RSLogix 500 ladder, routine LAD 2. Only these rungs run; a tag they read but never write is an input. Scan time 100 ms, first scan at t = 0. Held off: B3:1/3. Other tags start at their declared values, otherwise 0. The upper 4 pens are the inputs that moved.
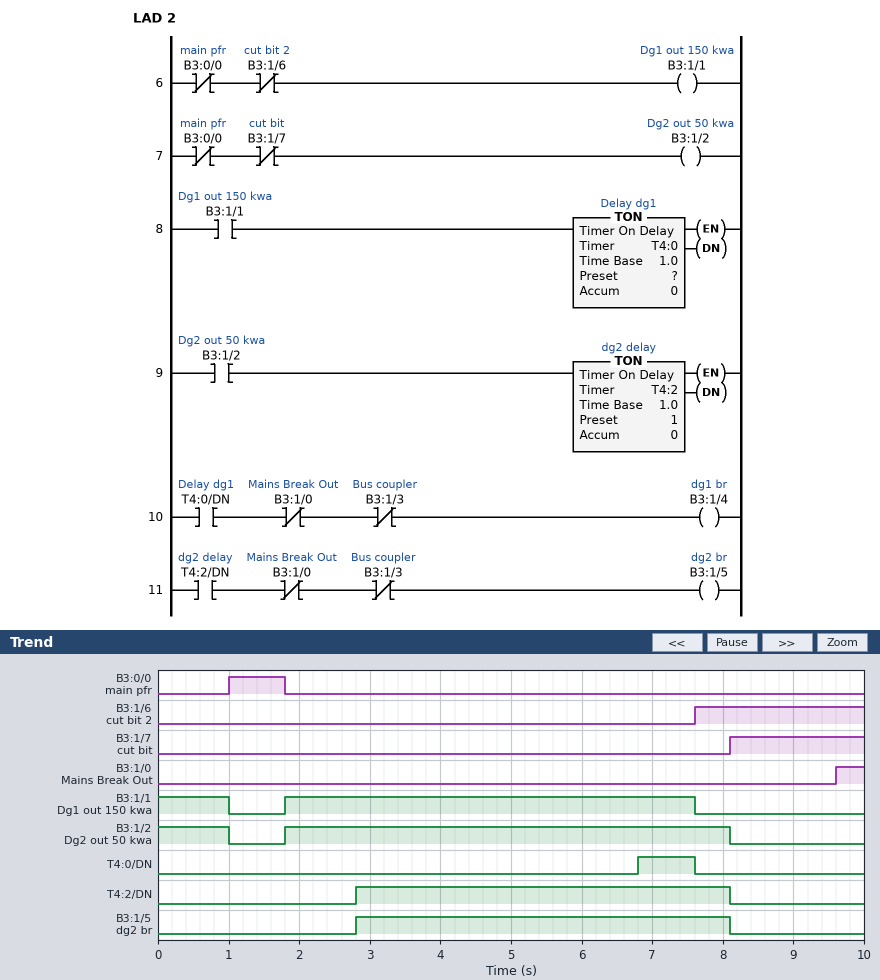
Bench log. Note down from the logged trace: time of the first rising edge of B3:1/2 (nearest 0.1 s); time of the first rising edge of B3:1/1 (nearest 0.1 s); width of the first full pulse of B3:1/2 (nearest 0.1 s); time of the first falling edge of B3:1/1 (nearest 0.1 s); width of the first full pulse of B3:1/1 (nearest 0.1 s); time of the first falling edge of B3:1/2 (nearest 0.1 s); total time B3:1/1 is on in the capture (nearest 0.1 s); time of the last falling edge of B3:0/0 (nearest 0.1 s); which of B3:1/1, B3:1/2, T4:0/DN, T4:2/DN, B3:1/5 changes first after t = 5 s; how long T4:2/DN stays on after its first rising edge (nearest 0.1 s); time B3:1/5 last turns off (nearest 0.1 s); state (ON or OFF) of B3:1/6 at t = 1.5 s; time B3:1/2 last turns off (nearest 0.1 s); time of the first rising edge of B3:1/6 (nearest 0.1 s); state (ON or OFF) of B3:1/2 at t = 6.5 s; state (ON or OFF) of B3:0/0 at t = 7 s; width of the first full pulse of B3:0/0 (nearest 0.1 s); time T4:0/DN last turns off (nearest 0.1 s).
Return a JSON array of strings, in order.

["1.8 s", "1.8 s", "6.3 s", "1.0 s", "5.8 s", "1.0 s", "6.8 s", "1.8 s", "T4:0/DN", "5.3 s", "8.1 s", "OFF", "8.1 s", "7.6 s", "ON", "OFF", "0.8 s", "7.6 s"]
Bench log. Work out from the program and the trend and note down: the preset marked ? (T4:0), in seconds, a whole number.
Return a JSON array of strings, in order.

["5 s"]
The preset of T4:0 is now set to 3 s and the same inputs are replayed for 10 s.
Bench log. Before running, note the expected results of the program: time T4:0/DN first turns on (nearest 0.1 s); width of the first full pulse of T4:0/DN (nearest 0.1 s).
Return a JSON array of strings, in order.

["4.8 s", "2.8 s"]
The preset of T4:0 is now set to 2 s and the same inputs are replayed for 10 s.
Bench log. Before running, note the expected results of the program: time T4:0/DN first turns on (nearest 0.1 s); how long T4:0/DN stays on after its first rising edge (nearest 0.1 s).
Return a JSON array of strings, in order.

["3.8 s", "3.8 s"]
